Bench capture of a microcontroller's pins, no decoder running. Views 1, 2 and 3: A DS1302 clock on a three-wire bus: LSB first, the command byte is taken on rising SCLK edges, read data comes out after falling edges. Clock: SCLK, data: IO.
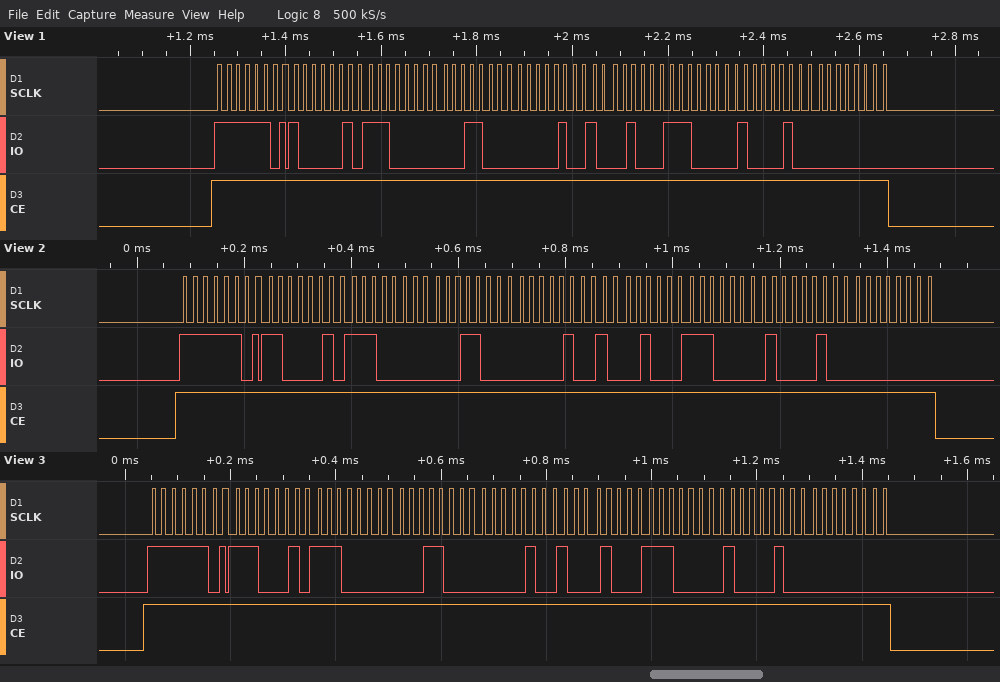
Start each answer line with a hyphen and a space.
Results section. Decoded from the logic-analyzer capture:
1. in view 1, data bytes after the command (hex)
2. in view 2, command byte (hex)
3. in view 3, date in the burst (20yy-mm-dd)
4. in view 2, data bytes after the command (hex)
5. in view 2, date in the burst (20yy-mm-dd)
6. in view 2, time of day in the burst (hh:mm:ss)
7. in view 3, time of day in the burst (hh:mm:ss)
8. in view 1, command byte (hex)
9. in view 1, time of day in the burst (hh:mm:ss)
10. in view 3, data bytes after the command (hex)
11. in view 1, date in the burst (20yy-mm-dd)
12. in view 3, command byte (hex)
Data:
- 41 07 18 20 11 07 21 00
- 0xBF
- 2021-11-20
- 43 07 18 20 11 07 21 00
- 2021-11-20
- 18:07:43
- 18:07:47
- 0xBF
- 18:07:41
- 47 07 18 20 11 07 21 00
- 2021-11-20
- 0xBF
